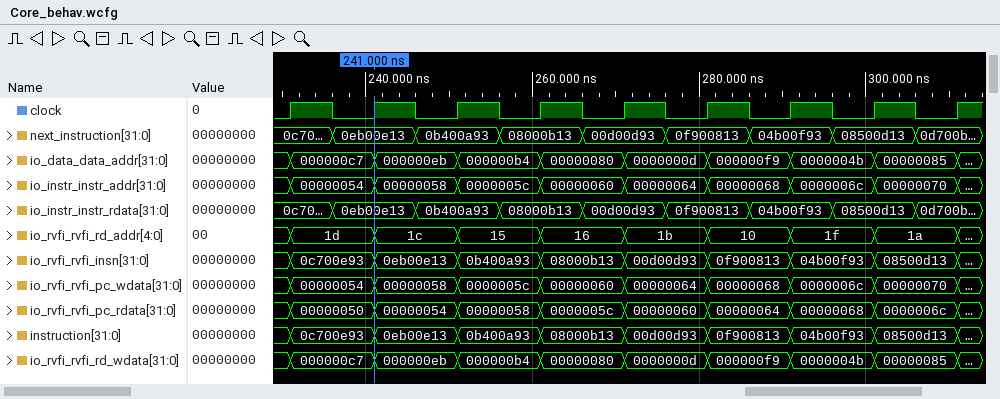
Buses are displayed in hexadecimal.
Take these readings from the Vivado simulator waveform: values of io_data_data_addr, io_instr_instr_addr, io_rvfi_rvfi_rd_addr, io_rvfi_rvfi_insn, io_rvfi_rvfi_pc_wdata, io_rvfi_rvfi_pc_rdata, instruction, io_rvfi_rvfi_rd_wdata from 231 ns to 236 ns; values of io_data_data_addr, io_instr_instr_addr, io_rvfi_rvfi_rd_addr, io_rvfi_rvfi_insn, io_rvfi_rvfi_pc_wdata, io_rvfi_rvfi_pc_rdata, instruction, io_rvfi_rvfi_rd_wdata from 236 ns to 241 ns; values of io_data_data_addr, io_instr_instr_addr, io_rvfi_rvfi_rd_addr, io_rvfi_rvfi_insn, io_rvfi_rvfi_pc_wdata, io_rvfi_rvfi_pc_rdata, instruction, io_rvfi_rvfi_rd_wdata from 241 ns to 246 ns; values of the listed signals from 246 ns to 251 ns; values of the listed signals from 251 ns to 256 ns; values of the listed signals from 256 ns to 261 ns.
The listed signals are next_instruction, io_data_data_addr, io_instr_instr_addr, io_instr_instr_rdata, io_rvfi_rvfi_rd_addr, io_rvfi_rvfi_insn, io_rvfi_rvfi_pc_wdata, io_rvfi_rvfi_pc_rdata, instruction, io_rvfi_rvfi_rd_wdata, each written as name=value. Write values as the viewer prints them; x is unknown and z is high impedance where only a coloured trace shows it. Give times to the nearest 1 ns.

io_data_data_addr=000000c7, io_instr_instr_addr=00000054, io_rvfi_rvfi_rd_addr=1d, io_rvfi_rvfi_insn=0c700e93, io_rvfi_rvfi_pc_wdata=00000054, io_rvfi_rvfi_pc_rdata=00000050, instruction=0c700e93, io_rvfi_rvfi_rd_wdata=000000c7
io_data_data_addr=000000c7, io_instr_instr_addr=00000054, io_rvfi_rvfi_rd_addr=1d, io_rvfi_rvfi_insn=0c700e93, io_rvfi_rvfi_pc_wdata=00000054, io_rvfi_rvfi_pc_rdata=00000050, instruction=0c700e93, io_rvfi_rvfi_rd_wdata=000000c7
io_data_data_addr=000000eb, io_instr_instr_addr=00000058, io_rvfi_rvfi_rd_addr=1c, io_rvfi_rvfi_insn=0eb00e13, io_rvfi_rvfi_pc_wdata=00000058, io_rvfi_rvfi_pc_rdata=00000054, instruction=0eb00e13, io_rvfi_rvfi_rd_wdata=000000eb
next_instruction=0b400a93, io_data_data_addr=000000eb, io_instr_instr_addr=00000058, io_instr_instr_rdata=0b400a93, io_rvfi_rvfi_rd_addr=1c, io_rvfi_rvfi_insn=0eb00e13, io_rvfi_rvfi_pc_wdata=00000058, io_rvfi_rvfi_pc_rdata=00000054, instruction=0eb00e13, io_rvfi_rvfi_rd_wdata=000000eb
next_instruction=0b400a93, io_data_data_addr=000000b4, io_instr_instr_addr=0000005c, io_instr_instr_rdata=0b400a93, io_rvfi_rvfi_rd_addr=15, io_rvfi_rvfi_insn=0b400a93, io_rvfi_rvfi_pc_wdata=0000005c, io_rvfi_rvfi_pc_rdata=00000058, instruction=0b400a93, io_rvfi_rvfi_rd_wdata=000000b4
next_instruction=08000b13, io_data_data_addr=000000b4, io_instr_instr_addr=0000005c, io_instr_instr_rdata=08000b13, io_rvfi_rvfi_rd_addr=15, io_rvfi_rvfi_insn=0b400a93, io_rvfi_rvfi_pc_wdata=0000005c, io_rvfi_rvfi_pc_rdata=00000058, instruction=0b400a93, io_rvfi_rvfi_rd_wdata=000000b4
